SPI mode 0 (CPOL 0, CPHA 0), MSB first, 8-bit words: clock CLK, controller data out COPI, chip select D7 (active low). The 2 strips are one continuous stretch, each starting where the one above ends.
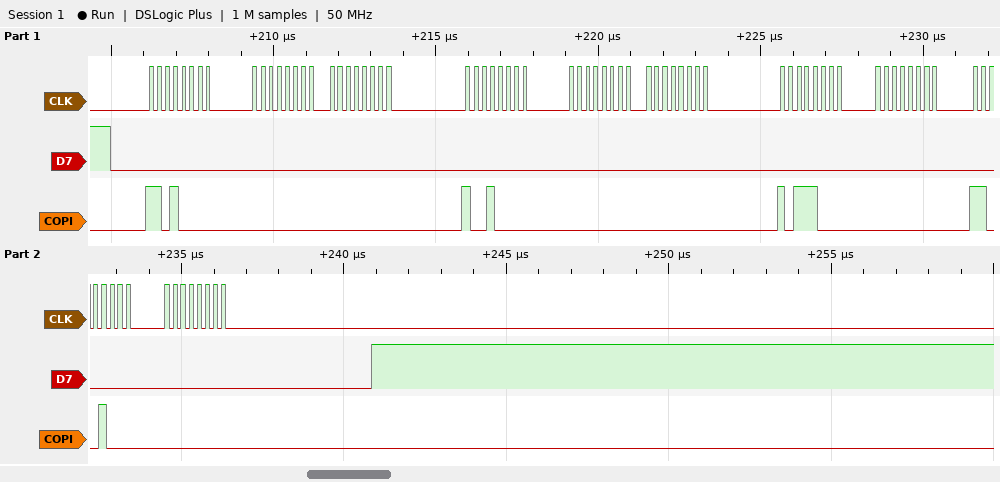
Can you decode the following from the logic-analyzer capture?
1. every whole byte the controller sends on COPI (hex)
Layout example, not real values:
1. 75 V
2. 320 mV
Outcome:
1. D0 00 00 90 00 00 B8 00 C8 00
